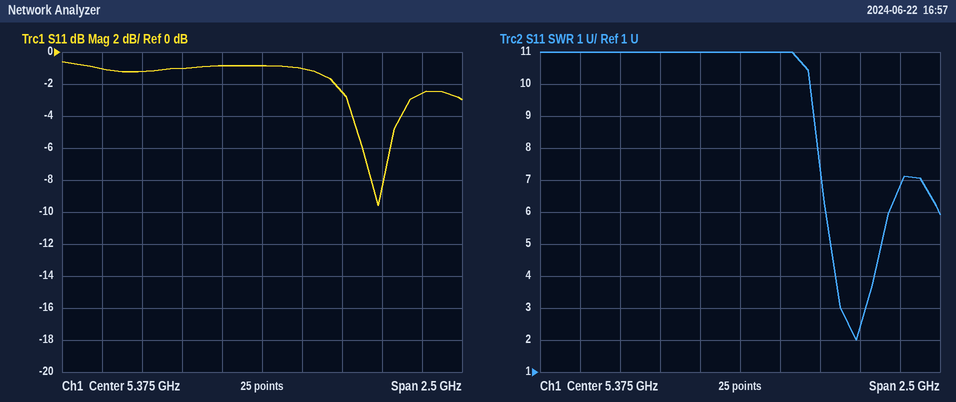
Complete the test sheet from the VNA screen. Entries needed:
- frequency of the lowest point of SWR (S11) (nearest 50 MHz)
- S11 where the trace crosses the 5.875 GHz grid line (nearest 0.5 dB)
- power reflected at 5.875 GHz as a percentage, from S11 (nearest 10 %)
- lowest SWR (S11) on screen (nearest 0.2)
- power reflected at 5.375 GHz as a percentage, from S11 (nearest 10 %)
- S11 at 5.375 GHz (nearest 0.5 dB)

6.10 GHz
-2.5 dB
60 %
2.0
80 %
-1.0 dB
